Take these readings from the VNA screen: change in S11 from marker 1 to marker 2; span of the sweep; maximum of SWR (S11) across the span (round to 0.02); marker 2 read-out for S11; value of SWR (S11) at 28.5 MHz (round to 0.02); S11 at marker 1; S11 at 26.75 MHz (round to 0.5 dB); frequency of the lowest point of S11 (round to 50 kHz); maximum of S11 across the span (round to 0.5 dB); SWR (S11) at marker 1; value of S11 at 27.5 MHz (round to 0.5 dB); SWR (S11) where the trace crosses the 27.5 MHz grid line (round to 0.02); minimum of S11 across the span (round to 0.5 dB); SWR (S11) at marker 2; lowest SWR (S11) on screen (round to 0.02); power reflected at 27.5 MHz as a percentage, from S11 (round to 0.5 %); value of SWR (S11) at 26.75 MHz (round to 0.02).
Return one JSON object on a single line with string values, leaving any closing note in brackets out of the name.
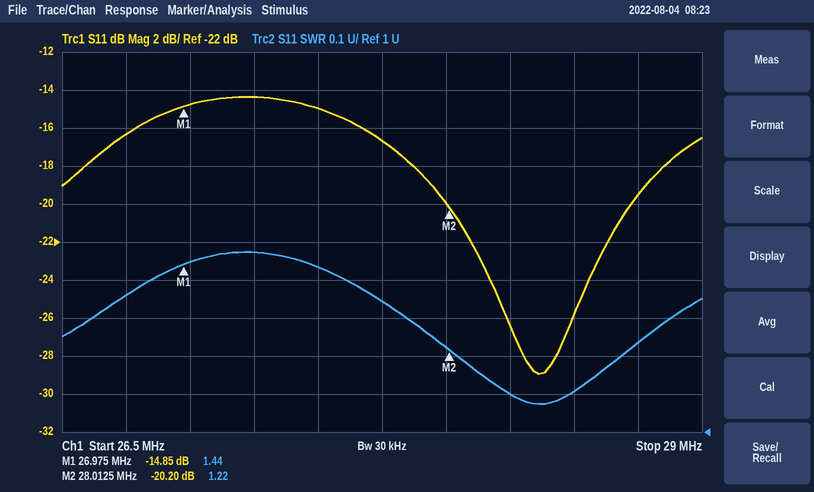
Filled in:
{"change in S11 from marker 1 to marker 2": "-5.35 dB", "span of the sweep": "2.5 MHz", "maximum of SWR (S11) across the span": "1.48", "marker 2 read-out for S11": "-20.20 dB", "value of SWR (S11) at 28.5 MHz": "1.10", "S11 at marker 1": "-14.85 dB", "S11 at 26.75 MHz": "-16.5 dB", "frequency of the lowest point of S11": "28.35 MHz", "maximum of S11 across the span": "-14.5 dB", "SWR (S11) at marker 1": "1.44", "value of S11 at 27.5 MHz": "-15.0 dB", "SWR (S11) where the trace crosses the 27.5 MHz grid line": "1.44", "minimum of S11 across the span": "-29.0 dB", "SWR (S11) at marker 2": "1.22", "lowest SWR (S11) on screen": "1.08", "power reflected at 27.5 MHz as a percentage, from S11": "3.0 %", "value of SWR (S11) at 26.75 MHz": "1.36"}
